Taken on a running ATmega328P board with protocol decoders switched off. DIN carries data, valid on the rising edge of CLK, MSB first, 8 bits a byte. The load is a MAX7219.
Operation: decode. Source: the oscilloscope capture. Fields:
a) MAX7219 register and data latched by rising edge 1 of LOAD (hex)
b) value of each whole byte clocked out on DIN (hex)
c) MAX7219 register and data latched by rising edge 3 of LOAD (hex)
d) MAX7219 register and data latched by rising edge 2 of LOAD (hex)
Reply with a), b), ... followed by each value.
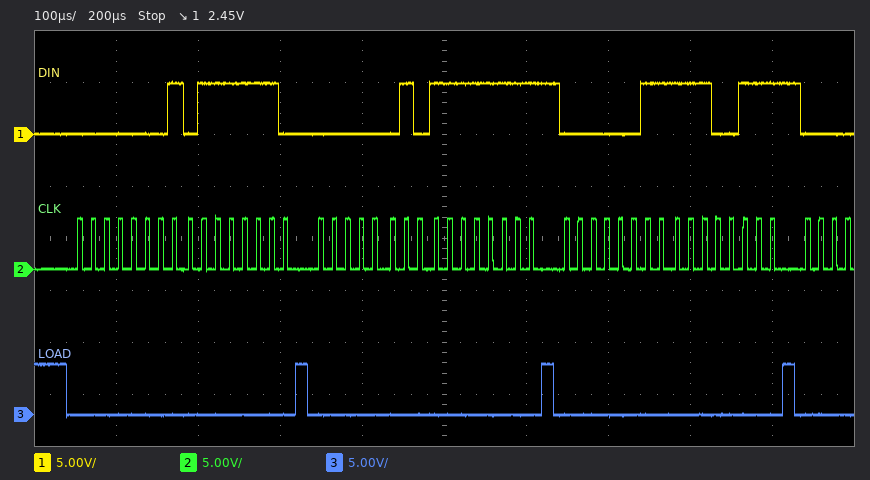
a) register 0x1, data 0x7E
b) 0x01 0x7E 0x02 0xFF 0x03 0xE7
c) register 0x3, data 0xE7
d) register 0x2, data 0xFF
